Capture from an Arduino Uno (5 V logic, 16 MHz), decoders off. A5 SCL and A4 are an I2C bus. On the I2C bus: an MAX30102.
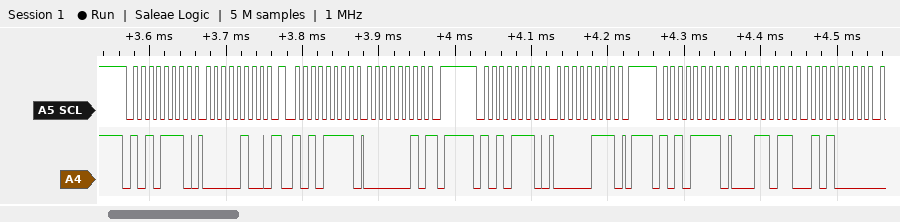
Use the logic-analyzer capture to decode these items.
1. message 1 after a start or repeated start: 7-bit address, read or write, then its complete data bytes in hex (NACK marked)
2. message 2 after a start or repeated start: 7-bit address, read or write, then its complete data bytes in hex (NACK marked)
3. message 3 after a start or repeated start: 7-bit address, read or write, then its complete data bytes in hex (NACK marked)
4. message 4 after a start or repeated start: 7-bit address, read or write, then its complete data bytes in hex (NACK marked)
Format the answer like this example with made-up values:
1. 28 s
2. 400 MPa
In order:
1. 0x57 write: 04
2. 0x57 read: 02 NACK
3. 0x57 write: 07
4. 0x57 read: 1B 50
